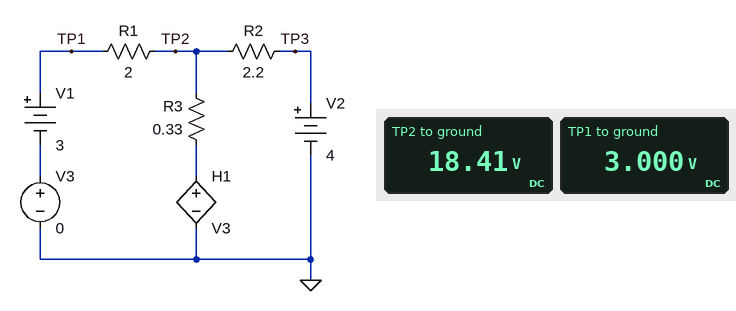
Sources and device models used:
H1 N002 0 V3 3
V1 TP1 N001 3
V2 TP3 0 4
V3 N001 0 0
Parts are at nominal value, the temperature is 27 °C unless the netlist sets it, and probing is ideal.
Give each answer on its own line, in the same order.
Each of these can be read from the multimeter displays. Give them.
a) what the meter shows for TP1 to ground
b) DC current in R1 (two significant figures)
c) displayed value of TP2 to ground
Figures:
3.000 V
7.7 A
18.41 V
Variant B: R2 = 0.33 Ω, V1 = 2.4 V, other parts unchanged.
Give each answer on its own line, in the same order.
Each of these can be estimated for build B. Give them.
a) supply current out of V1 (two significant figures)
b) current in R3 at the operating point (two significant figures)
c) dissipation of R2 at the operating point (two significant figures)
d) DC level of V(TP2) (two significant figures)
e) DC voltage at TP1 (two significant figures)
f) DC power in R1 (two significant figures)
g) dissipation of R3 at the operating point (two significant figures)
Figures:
600 mA
9.1 A
24 W
1.2 V
2.4 V
720 mW
27 W
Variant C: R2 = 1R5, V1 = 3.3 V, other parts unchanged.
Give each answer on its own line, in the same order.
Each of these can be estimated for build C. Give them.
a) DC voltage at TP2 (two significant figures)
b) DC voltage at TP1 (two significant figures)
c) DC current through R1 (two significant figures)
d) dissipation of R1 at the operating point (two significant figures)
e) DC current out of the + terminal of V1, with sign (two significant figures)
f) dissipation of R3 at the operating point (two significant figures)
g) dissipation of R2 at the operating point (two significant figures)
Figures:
31 V
3.3 V
14 A
370 W
-14 A
330 W
470 W
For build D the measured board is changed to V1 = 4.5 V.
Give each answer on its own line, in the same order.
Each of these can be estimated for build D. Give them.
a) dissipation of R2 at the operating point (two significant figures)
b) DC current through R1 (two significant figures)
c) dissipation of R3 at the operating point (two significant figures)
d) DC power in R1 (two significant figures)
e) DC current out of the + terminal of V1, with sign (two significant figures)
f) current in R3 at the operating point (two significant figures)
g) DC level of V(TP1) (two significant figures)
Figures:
290 W
12 A
190 W
310 W
-12 A
24 A
4.5 V
